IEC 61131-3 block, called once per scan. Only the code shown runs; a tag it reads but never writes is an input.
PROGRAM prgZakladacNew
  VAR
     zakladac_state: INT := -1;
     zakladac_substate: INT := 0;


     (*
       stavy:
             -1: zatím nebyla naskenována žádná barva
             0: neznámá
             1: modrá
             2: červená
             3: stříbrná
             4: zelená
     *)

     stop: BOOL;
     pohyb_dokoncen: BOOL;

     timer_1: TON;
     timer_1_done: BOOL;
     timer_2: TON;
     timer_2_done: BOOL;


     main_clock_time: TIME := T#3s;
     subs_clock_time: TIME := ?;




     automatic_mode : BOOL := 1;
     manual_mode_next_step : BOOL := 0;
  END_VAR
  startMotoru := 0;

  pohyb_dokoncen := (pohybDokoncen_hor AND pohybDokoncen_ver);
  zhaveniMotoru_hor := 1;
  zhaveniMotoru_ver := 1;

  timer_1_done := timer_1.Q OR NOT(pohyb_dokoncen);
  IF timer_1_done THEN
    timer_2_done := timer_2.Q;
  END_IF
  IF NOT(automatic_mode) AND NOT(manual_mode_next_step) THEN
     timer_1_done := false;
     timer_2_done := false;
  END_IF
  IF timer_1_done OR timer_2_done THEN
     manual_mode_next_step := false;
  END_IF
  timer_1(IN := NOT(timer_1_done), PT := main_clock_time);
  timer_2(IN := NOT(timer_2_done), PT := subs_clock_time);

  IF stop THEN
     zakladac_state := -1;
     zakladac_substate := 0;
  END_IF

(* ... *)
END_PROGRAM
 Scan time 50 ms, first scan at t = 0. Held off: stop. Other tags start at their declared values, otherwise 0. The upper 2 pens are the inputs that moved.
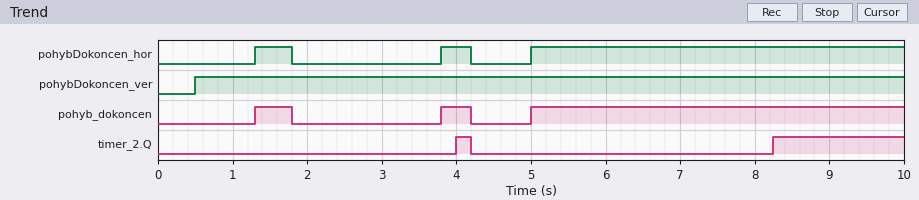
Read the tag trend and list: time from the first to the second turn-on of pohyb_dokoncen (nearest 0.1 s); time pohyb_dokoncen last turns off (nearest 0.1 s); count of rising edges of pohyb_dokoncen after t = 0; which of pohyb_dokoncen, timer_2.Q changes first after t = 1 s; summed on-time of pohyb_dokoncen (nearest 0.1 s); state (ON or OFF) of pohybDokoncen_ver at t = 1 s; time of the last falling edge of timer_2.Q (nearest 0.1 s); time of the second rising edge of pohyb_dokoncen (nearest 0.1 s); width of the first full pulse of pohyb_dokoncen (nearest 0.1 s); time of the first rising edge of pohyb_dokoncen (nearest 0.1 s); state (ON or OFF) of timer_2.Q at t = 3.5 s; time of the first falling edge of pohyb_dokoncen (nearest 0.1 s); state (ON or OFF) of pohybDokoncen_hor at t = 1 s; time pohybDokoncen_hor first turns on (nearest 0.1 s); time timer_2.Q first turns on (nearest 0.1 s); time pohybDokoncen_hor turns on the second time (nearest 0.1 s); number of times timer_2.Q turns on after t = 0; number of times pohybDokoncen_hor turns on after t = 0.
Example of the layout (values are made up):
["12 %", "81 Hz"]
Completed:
["2.5 s", "4.2 s", "3", "pohyb_dokoncen", "5.9 s", "ON", "4.2 s", "3.8 s", "0.5 s", "1.3 s", "OFF", "1.8 s", "OFF", "1.3 s", "4.0 s", "3.8 s", "2", "3"]
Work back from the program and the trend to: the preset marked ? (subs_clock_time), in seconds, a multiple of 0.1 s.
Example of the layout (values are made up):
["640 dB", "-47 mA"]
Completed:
["4.0 s"]
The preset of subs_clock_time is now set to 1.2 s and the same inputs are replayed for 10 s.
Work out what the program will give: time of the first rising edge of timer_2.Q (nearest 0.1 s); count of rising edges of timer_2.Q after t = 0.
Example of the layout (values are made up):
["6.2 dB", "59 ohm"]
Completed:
["1.2 s", "4"]
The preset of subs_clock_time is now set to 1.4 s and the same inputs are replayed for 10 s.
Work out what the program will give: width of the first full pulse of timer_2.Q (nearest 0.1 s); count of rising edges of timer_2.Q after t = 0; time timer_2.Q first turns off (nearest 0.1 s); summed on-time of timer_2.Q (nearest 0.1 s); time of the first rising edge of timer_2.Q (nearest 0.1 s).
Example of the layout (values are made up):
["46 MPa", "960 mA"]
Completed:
["0.4 s", "4", "1.8 s", "2.3 s", "1.4 s"]
